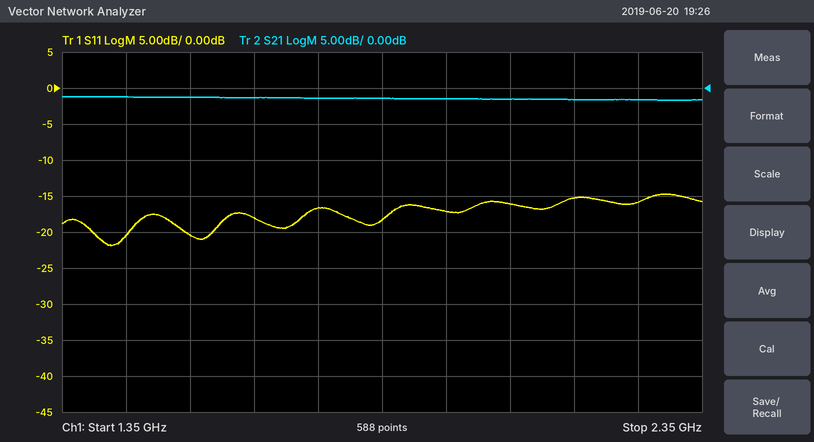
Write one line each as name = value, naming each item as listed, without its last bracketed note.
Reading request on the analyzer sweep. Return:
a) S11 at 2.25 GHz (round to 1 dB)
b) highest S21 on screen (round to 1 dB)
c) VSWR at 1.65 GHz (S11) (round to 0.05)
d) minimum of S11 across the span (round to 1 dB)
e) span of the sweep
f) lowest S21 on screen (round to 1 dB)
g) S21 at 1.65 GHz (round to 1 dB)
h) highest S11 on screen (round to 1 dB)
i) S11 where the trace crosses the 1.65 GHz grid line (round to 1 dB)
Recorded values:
S11 at 2.25 GHz = -16 dB
highest S21 on screen = -1 dB
VSWR at 1.65 GHz (S11) = 1.30
minimum of S11 across the span = -22 dB
span of the sweep = 1 GHz
lowest S21 on screen = -2 dB
S21 at 1.65 GHz = -1 dB
highest S11 on screen = -15 dB
S11 where the trace crosses the 1.65 GHz grid line = -18 dB
